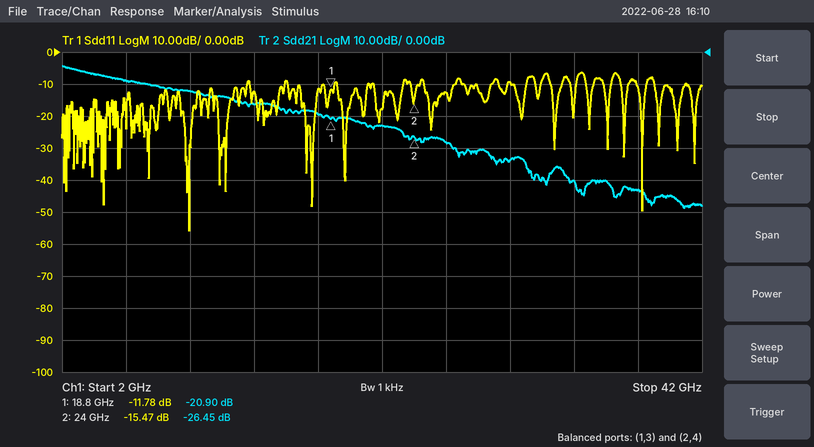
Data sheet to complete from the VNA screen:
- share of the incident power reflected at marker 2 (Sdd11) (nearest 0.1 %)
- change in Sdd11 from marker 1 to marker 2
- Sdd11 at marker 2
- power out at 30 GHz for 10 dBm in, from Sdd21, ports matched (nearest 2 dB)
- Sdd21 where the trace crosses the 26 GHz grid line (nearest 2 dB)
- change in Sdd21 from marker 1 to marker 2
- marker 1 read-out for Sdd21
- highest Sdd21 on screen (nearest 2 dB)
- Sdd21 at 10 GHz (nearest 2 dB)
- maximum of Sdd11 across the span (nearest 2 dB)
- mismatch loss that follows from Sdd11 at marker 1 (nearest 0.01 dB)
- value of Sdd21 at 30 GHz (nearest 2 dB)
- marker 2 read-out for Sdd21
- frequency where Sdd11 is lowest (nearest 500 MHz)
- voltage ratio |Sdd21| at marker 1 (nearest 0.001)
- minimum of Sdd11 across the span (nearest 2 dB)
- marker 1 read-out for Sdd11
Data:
2.8 %
-3.69 dB
-15.47 dB
-24 dBm
-28 dB
-5.55 dB
-20.90 dB
-4 dB
-12 dB
-6 dB
0.30 dB
-34 dB
-26.45 dB
10.0 GHz
0.090
-56 dB
-11.78 dB
